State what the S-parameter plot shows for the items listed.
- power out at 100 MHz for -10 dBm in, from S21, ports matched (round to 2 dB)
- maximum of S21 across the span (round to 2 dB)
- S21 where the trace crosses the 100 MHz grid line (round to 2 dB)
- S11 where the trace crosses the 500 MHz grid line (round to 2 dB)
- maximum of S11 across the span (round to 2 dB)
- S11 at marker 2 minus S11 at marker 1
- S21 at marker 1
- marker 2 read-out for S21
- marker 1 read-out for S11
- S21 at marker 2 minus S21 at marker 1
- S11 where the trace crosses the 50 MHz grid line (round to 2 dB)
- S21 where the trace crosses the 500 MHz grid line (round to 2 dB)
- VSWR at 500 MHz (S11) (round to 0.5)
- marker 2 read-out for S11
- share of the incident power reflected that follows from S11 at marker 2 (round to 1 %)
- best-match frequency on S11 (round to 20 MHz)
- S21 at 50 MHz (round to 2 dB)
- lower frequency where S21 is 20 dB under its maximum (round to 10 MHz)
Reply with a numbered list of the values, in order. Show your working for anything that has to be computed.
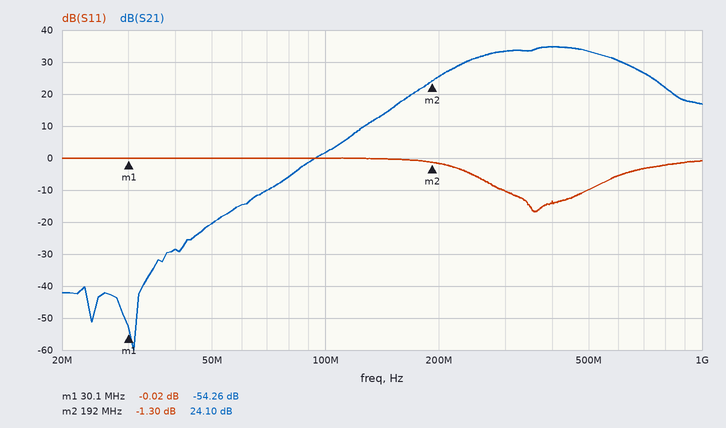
1. -10 dBm + (2 dB) = -8 dBm
2. 34 dB
3. 2 dB
4. -10 dB
5. 0 dB
6. -1.3 − (-0.02) = -1.28 dB
7. -54.26 dB
8. 24.10 dB
9. -0.02 dB
10. 24.1 − (-54.26) = 78.36 dB
11. 0 dB
12. 34 dB
13. |Γ| = 10^(-10/20) = 0.3162; VSWR = (1 + 0.3162)/(1 − 0.3162) ≈ 1.92, so 2.0 to the nearest 0.5
14. -1.30 dB
15. 10^(-1.3/10) ≈ 74 %
16. 360 MHz
17. -20 dB
18. 150 MHz
